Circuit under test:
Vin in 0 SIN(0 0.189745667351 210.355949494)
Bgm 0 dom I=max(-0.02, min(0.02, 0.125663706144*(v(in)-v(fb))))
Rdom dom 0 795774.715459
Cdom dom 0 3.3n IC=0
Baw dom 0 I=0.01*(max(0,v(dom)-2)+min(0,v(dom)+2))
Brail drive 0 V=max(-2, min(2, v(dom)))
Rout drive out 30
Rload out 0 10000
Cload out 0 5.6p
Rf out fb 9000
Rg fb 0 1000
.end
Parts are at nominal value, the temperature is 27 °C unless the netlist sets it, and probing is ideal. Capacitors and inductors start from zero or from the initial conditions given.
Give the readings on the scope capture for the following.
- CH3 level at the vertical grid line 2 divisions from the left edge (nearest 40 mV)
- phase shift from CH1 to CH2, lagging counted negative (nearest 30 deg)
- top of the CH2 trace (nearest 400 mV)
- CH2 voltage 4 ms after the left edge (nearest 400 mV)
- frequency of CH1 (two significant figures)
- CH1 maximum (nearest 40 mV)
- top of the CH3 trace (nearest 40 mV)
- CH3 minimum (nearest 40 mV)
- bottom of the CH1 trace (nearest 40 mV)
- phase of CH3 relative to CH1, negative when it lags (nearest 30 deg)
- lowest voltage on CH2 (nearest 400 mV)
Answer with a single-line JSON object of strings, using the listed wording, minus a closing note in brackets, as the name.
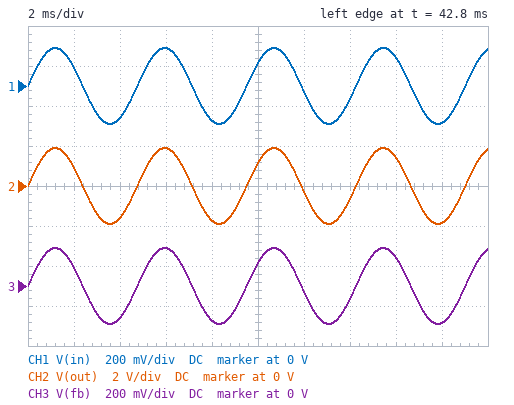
{"CH3 level at the vertical grid line 2 divisions from the left edge": "-160 mV", "phase shift from CH1 to CH2, lagging counted negative": "0 deg", "top of the CH2 trace": "2.0 V", "CH2 voltage 4 ms after the left edge": "-1.6 V", "frequency of CH1": "210 Hz", "CH1 maximum": "200 mV", "top of the CH3 trace": "200 mV", "CH3 minimum": "-200 mV", "bottom of the CH1 trace": "-200 mV", "phase of CH3 relative to CH1, negative when it lags": "0 deg", "lowest voltage on CH2": "-2.0 V"}
